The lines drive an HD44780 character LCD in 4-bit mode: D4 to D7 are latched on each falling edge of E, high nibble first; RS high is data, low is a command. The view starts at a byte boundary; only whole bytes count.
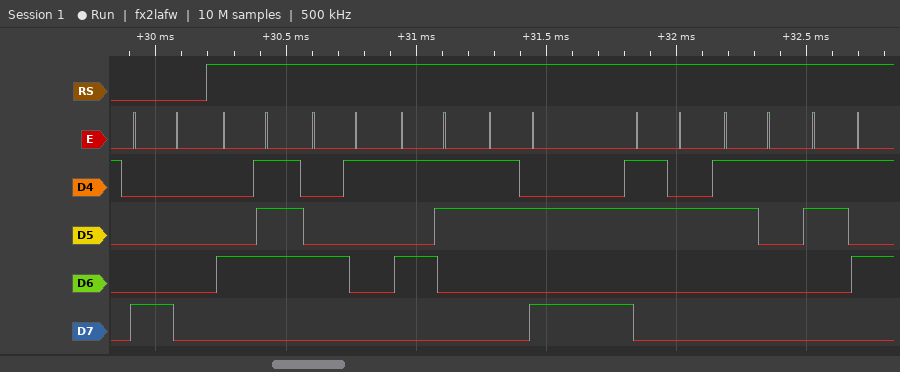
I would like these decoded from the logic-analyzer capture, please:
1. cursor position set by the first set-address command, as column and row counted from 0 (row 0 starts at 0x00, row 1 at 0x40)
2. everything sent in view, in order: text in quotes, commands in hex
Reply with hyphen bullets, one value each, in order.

- column 0, row 0
- 0x80 "GAS:215"
